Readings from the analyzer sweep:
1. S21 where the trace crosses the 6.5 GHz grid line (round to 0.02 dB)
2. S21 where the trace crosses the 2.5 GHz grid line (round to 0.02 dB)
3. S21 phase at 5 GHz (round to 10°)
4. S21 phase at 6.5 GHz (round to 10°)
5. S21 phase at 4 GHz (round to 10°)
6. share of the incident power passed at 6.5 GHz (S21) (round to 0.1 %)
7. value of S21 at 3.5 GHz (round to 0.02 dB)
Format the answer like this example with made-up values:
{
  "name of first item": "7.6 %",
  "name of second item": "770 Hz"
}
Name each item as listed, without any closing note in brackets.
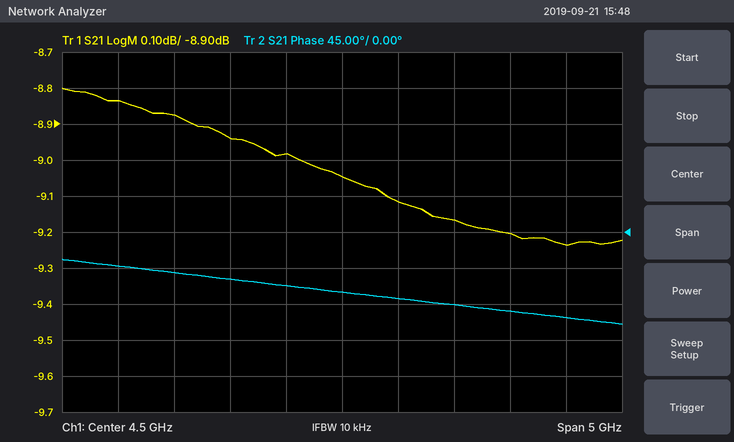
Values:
{
  "S21 where the trace crosses the 6.5 GHz grid line": "-9.24 dB",
  "S21 where the trace crosses the 2.5 GHz grid line": "-8.84 dB",
  "S21 phase at 5 GHz": "-80°",
  "S21 phase at 6.5 GHz": "-110°",
  "S21 phase at 4 GHz": "-70°",
  "share of the incident power passed at 6.5 GHz (S21)": "11.9 %",
  "value of S21 at 3.5 GHz": "-8.94 dB"
}
